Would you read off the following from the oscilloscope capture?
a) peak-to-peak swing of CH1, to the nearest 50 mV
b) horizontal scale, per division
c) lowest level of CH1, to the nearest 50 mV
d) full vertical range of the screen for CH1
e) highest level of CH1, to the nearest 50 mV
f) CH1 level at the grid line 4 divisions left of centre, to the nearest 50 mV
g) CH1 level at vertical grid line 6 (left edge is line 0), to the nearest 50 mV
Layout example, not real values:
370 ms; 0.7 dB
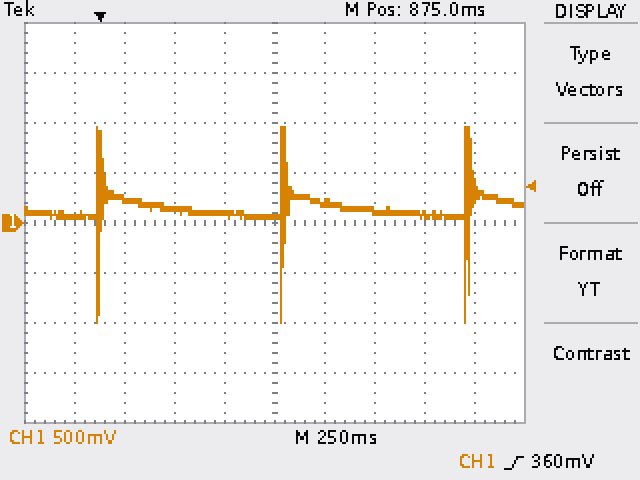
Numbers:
1.95 V; 250 ms; -1.00 V; 4 V; 950 mV; 50 mV; 200 mV
